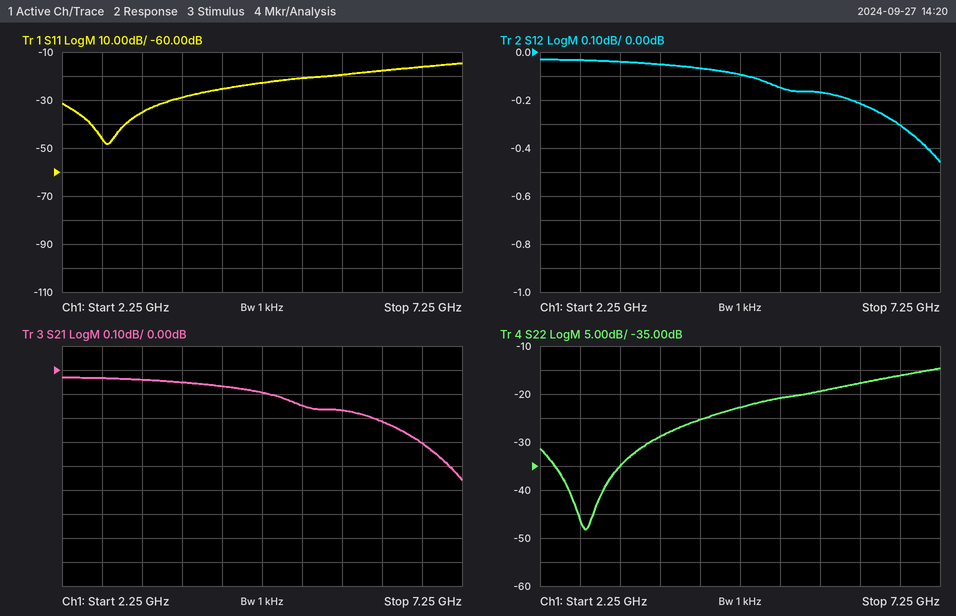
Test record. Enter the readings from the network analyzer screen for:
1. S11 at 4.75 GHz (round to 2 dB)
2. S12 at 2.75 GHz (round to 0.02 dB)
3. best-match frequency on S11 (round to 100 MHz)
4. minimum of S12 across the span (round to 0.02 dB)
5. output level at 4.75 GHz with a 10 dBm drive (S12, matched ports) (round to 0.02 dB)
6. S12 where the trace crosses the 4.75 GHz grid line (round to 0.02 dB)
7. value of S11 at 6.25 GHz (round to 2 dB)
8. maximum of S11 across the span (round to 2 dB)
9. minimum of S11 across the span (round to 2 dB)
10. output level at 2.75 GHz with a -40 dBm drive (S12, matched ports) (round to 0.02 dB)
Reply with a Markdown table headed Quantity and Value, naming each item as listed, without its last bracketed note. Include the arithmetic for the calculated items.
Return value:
| Quantity | Value |
|---|---|
| S11 at 4.75 GHz | -22 dB |
| S12 at 2.75 GHz | -0.04 dB |
| best-match frequency on S11 | 2.8 GHz |
| minimum of S12 across the span | -0.46 dB |
| output level at 4.75 GHz with a 10 dBm drive (S12, matched ports) | 10 dBm + (-0.10 dB) = 9.90 dBm |
| S12 where the trace crosses the 4.75 GHz grid line | -0.10 dB |
| value of S11 at 6.25 GHz | -18 dB |
| maximum of S11 across the span | -14 dB |
| minimum of S11 across the span | -48 dB |
| output level at 2.75 GHz with a -40 dBm drive (S12, matched ports) | -40 dBm + (-0.04 dB) = -40.04 dBm |
